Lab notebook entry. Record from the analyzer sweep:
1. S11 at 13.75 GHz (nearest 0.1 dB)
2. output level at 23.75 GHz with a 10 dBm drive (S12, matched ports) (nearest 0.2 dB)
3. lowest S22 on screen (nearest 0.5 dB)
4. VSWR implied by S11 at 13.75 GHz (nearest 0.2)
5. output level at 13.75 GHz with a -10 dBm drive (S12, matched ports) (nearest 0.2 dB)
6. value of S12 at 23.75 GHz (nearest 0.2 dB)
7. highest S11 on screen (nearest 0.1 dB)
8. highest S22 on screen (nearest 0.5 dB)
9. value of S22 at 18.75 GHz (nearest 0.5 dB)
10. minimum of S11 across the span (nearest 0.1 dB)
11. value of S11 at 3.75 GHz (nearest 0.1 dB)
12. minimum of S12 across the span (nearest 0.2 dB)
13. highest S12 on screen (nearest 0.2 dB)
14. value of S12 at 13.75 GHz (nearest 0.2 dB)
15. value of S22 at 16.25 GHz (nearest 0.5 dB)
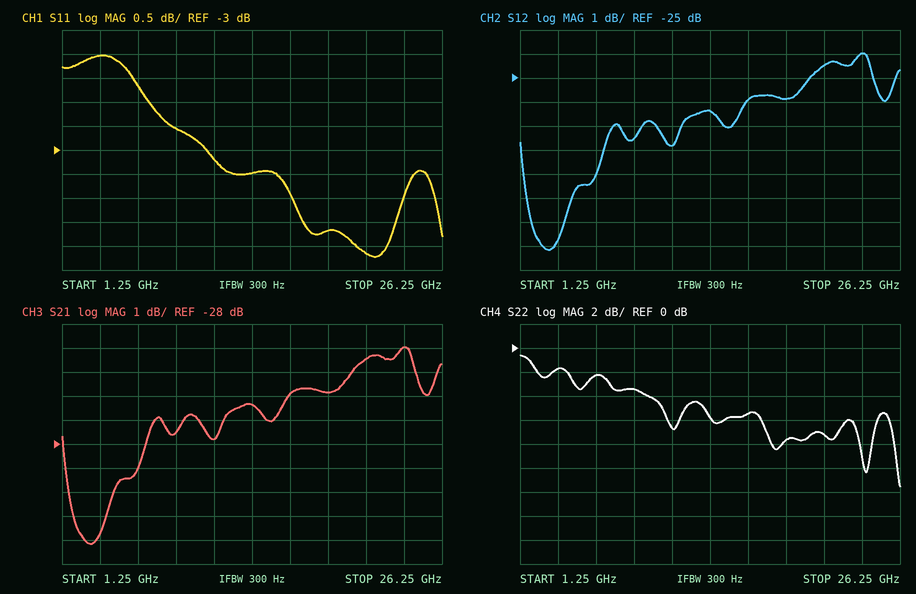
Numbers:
-3.5 dB
-14.0 dBm
-11.5 dB
5.0
-36.4 dBm
-24.0 dB
-1.0 dB
-0.5 dB
-7.5 dB
-5.2 dB
-1.0 dB
-32.2 dB
-24.0 dB
-26.4 dB
-5.5 dB
